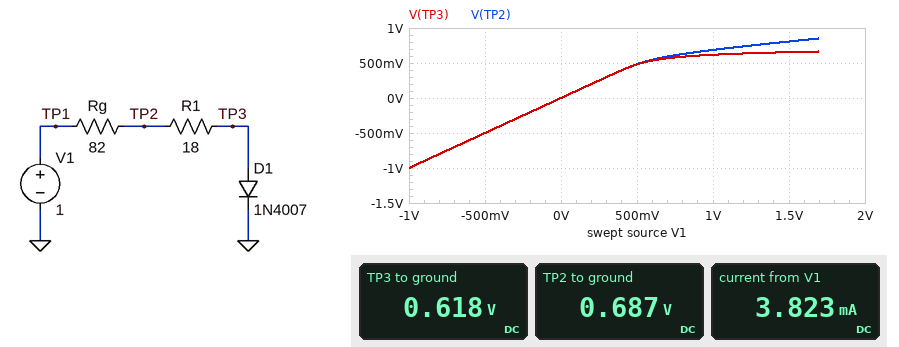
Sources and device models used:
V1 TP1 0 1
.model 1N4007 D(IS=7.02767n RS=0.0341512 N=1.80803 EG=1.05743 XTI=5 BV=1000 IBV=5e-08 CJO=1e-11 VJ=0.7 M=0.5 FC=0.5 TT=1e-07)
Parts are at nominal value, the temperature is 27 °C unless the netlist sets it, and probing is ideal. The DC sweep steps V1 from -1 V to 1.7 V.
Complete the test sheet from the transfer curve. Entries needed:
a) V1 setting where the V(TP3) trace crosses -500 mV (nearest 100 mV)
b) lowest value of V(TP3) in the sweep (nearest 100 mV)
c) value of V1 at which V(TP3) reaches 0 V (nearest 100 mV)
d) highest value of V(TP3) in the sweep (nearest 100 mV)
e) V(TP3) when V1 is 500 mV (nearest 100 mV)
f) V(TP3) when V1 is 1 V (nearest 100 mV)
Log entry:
-500 mV
-1.0 V
0 V
700 mV
500 mV
600 mV
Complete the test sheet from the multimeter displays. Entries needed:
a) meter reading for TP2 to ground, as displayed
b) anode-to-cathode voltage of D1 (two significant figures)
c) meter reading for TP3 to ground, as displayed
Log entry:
0.687 V
620 mV
0.618 V
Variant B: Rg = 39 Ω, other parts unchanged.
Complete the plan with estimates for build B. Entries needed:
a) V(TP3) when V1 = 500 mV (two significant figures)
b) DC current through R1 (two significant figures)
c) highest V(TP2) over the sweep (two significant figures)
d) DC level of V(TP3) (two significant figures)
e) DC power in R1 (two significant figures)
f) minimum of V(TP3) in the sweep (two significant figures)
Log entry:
490 mV
6.3 mA
1.0 V
640 mV
710 µW
-1.0 V
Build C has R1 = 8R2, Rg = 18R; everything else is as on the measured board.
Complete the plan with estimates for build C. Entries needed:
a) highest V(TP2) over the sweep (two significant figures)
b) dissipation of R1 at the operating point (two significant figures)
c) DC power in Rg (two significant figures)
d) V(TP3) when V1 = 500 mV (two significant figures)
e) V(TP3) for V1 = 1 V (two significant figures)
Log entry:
1.0 V
1.3 mW
2.8 mW
490 mV
670 mV
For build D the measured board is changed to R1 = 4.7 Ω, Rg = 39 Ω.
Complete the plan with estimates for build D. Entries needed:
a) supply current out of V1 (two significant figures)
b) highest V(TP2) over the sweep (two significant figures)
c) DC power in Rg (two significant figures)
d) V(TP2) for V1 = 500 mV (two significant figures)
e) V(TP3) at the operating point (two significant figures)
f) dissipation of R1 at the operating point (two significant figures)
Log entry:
8.0 mA
810 mV
2.5 mW
490 mV
650 mV
300 µW
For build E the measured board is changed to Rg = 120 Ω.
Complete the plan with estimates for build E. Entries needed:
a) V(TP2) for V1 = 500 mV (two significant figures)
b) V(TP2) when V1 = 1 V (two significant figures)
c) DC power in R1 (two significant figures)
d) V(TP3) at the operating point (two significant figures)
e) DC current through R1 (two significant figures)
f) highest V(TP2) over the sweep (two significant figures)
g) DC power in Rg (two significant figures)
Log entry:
480 mV
660 mV
150 µW
600 mV
2.9 mA
790 mV
990 µW
